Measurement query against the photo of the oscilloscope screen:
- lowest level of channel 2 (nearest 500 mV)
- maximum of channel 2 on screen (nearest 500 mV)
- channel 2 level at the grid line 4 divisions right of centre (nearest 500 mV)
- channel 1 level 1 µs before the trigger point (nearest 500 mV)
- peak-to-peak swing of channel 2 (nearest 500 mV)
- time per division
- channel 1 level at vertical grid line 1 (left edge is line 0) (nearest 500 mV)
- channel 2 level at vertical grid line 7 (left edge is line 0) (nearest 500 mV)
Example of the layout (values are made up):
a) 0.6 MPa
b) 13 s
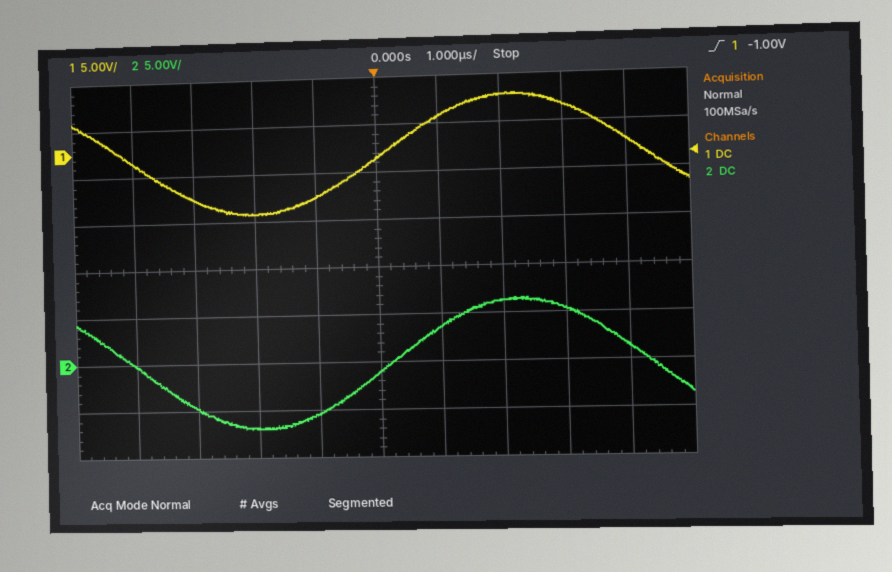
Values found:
a) -7.0 V
b) 6.5 V
c) 1.5 V
d) -5.0 V
e) 13.5 V
f) 1 µs
g) -1.0 V
h) 6.5 V
